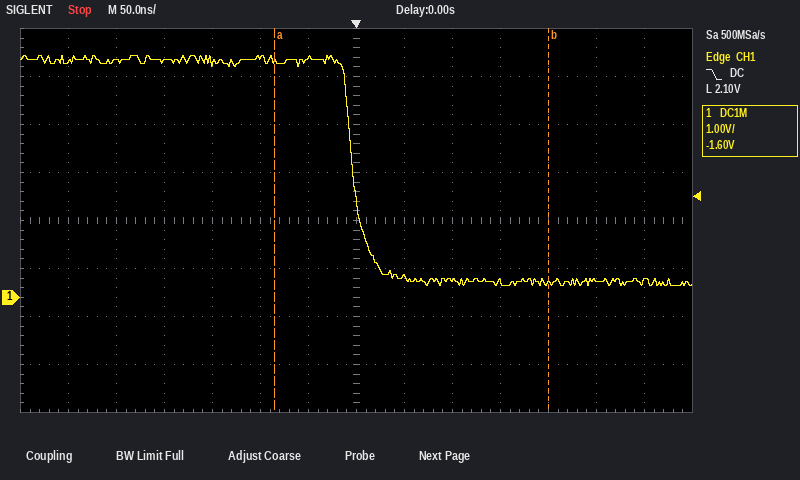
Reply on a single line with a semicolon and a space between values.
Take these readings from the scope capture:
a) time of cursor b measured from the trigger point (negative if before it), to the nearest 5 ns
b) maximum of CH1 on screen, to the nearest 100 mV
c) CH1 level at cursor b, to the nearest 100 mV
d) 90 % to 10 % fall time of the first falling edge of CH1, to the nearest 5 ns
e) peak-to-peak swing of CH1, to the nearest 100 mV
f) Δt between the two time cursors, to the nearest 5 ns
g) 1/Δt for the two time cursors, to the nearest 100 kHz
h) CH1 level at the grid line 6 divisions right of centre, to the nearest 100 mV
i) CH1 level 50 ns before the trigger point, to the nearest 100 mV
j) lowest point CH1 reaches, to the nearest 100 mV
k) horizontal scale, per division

+200 ns; 5.0 V; 300 mV; 30 ns; 4.8 V; 285 ns; 3.5 MHz; 300 mV; 5.0 V; 200 mV; 50 ns
